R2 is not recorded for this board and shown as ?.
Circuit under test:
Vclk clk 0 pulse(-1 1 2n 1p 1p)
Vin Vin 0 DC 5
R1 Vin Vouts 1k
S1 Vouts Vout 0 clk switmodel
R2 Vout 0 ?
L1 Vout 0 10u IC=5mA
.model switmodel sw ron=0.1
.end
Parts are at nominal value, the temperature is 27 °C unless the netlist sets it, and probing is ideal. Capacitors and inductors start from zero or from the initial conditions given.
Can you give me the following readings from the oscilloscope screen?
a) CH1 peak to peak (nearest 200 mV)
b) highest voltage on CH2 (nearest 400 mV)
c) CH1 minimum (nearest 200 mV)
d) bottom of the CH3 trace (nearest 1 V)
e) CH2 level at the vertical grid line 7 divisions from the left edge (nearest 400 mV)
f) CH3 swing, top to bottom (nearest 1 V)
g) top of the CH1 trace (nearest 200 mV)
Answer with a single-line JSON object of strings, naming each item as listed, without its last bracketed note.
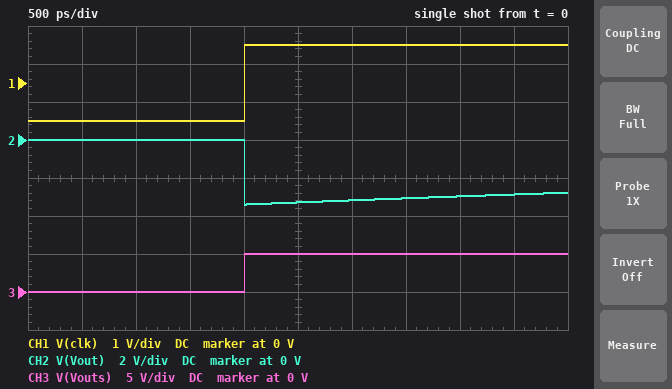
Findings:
{"CH1 peak to peak": "2.0 V", "highest voltage on CH2": "0 V", "CH1 minimum": "-1.0 V", "bottom of the CH3 trace": "0 V", "CH2 level at the vertical grid line 7 divisions from the left edge": "-3.2 V", "CH3 swing, top to bottom": "5 V", "top of the CH1 trace": "1.0 V"}
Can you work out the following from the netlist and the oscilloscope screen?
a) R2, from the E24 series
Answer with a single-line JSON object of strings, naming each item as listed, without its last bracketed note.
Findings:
{"R2, from the E24 series": "680 Ω"}
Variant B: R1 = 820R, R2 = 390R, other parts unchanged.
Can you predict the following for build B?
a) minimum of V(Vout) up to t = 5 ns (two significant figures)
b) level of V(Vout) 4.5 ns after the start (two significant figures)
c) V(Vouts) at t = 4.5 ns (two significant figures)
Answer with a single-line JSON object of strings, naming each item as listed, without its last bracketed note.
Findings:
{"minimum of V(Vout) up to t = 5 ns": "-2.0 V", "level of V(Vout) 4.5 ns after the start": "-1.8 V", "V(Vouts) at t = 4.5 ns": "5.0 V"}
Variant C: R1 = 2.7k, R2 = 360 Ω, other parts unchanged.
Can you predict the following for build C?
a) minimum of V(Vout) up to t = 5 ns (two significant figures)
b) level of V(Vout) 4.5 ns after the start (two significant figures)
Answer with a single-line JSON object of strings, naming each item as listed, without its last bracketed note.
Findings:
{"minimum of V(Vout) up to t = 5 ns": "-1.7 V", "level of V(Vout) 4.5 ns after the start": "-1.6 V"}
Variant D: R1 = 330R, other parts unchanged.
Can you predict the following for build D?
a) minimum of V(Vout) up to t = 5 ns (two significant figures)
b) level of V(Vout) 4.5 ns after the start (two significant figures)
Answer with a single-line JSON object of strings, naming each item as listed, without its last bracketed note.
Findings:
{"minimum of V(Vout) up to t = 5 ns": "-3.7 V", "level of V(Vout) 4.5 ns after the start": "-3.1 V"}
